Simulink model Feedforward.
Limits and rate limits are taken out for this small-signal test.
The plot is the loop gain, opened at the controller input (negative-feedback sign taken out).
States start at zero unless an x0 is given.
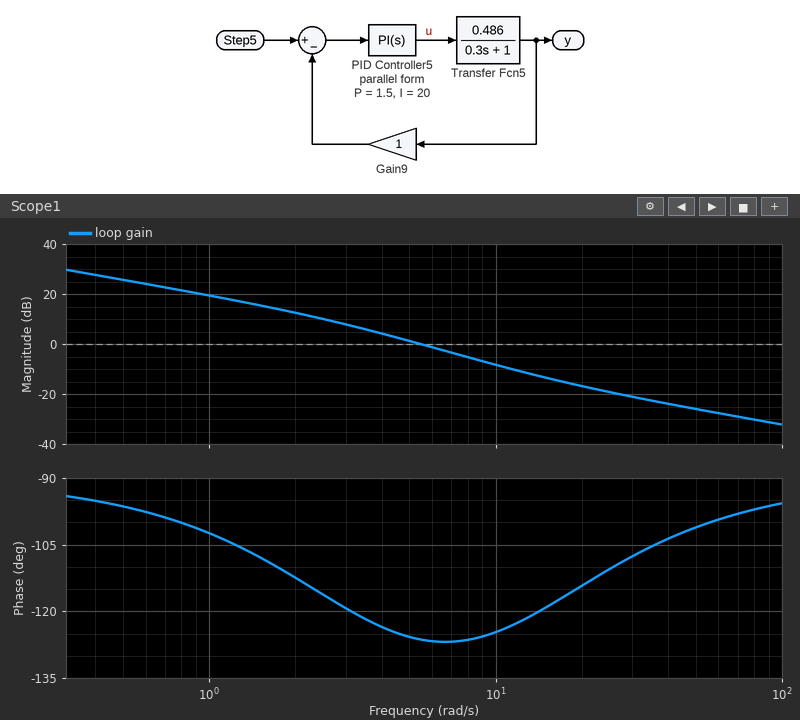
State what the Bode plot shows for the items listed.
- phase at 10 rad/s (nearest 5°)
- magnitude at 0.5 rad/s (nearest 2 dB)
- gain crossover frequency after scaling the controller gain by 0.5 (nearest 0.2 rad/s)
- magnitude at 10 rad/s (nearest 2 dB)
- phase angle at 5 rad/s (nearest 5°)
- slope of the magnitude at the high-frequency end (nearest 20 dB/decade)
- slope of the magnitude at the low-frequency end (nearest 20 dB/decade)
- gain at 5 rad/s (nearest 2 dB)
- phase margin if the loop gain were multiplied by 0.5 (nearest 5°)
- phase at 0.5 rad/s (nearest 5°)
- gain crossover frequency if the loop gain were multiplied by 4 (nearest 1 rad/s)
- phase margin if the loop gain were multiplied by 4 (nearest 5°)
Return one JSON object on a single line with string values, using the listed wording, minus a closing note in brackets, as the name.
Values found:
{"phase at 10 rad/s": "-125°", "magnitude at 0.5 rad/s": "26 dB", "gain crossover frequency after scaling the controller gain by 0.5": "3.4 rad/s", "magnitude at 10 rad/s": "-8 dB", "phase angle at 5 rad/s": "-125°", "slope of the magnitude at the high-frequency end": "-20 dB/decade", "slope of the magnitude at the low-frequency end": "-20 dB/decade", "gain at 5 rad/s": "2 dB", "phase margin if the loop gain were multiplied by 0.5": "60°", "phase at 0.5 rad/s": "-95°", "gain crossover frequency if the loop gain were multiplied by 4": "13 rad/s", "phase margin if the loop gain were multiplied by 4": "60°"}
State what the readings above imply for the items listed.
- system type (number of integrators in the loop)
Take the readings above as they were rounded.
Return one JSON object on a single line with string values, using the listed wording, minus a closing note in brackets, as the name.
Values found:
{"system type": "1"}
